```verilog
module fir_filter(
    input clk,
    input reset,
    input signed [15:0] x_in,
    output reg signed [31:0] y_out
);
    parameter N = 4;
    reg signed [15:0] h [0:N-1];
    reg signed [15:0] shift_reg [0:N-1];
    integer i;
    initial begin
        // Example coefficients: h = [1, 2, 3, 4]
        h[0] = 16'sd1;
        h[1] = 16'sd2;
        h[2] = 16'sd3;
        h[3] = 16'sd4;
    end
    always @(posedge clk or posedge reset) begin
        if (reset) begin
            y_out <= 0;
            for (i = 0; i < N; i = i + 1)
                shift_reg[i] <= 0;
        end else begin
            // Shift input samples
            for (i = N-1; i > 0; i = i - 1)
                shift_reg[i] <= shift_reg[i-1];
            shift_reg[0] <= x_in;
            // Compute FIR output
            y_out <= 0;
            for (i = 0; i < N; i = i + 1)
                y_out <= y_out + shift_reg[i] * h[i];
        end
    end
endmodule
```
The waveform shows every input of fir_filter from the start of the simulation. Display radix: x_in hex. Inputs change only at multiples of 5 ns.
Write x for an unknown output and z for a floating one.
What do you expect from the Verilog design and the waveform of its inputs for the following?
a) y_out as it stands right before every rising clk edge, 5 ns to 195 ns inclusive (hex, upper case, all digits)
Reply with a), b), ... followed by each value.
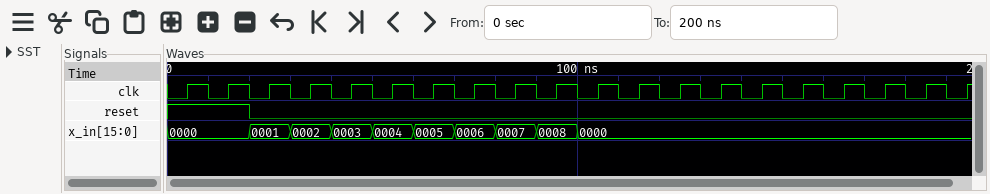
a) 00000000, 00000000, 00000000, 00000000, 00000000, 00000000, 00000000, 00000004, 0000000C, 00000018, 00000028, 0000003C, 00000054, 00000070, 00000090, 00000090, 00000090, 00000090, 00000090, 00000090
